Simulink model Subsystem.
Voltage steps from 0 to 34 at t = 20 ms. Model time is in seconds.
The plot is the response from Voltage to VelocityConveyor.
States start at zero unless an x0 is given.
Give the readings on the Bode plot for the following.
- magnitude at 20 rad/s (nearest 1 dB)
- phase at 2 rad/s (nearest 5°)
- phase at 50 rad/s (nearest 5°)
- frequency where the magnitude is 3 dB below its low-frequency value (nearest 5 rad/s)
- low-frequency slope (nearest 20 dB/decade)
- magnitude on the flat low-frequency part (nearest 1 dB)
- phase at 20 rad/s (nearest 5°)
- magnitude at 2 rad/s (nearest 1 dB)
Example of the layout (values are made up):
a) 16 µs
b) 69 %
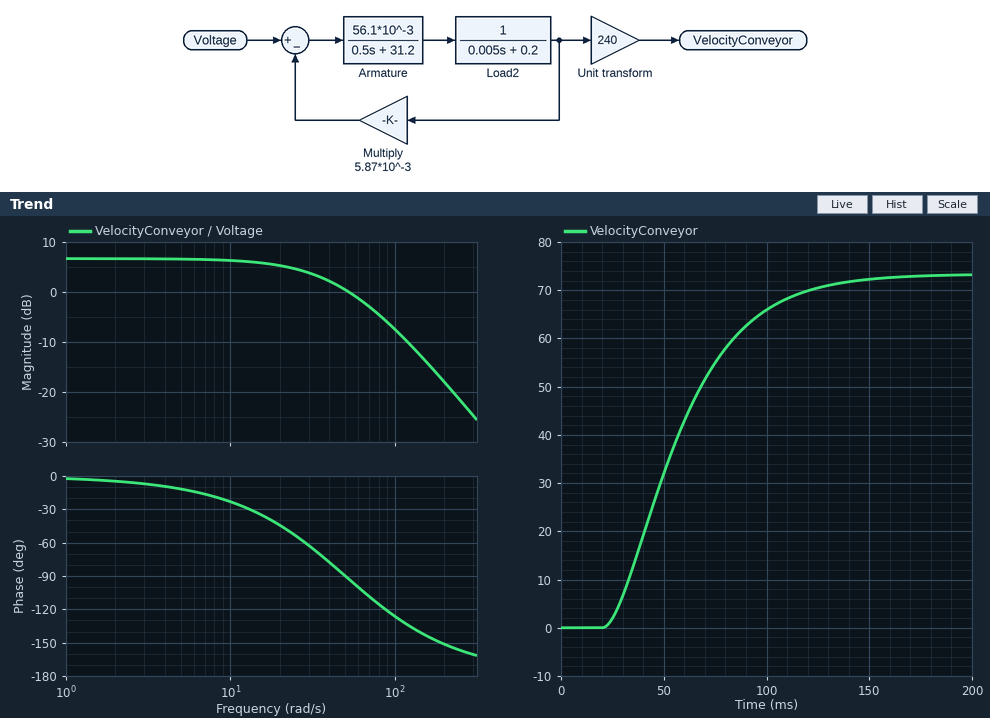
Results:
a) 5 dB
b) -5°
c) -90°
d) 30 rad/s
e) 0 dB/decade
f) 7 dB
g) -45°
h) 7 dB
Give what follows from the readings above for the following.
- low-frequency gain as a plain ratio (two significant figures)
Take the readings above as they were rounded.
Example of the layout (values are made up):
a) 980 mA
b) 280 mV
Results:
a) 2.2
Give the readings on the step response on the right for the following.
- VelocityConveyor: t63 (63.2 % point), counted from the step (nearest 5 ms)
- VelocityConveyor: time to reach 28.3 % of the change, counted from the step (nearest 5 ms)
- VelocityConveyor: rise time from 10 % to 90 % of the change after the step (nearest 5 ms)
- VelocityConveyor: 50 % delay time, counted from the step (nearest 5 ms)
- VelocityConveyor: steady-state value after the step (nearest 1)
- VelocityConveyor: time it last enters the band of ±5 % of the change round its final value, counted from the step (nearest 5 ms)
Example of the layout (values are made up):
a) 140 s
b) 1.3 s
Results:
a) 45 ms
b) 20 ms
c) 70 ms
d) 35 ms
e) 73
f) 100 ms
